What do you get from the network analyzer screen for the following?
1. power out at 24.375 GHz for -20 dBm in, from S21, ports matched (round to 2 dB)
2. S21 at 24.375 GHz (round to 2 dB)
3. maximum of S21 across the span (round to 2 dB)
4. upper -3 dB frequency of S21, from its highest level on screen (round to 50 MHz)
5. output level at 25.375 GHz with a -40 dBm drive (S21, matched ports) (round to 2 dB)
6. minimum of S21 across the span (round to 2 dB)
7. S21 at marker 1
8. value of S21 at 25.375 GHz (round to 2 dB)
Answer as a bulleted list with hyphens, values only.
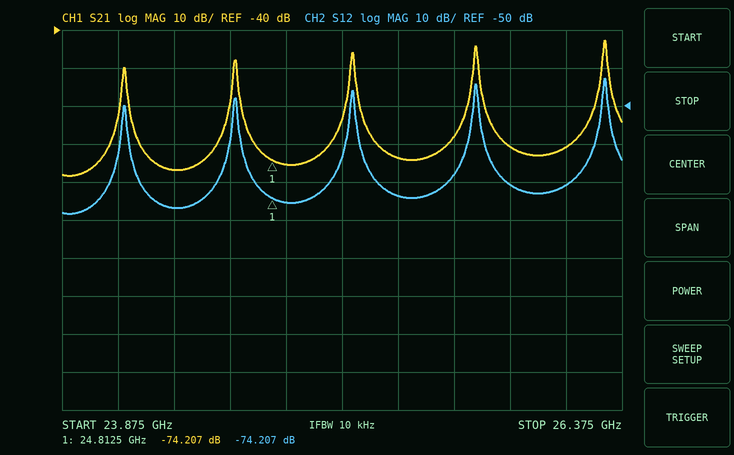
- -96 dBm
- -76 dB
- -42 dB
- 26.30 GHz
- -114 dBm
- -78 dB
- -74.207 dB
- -74 dB
